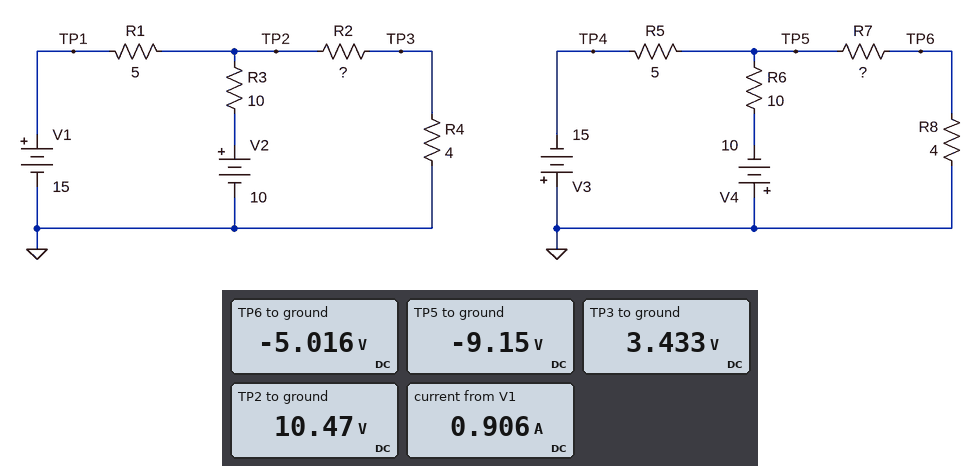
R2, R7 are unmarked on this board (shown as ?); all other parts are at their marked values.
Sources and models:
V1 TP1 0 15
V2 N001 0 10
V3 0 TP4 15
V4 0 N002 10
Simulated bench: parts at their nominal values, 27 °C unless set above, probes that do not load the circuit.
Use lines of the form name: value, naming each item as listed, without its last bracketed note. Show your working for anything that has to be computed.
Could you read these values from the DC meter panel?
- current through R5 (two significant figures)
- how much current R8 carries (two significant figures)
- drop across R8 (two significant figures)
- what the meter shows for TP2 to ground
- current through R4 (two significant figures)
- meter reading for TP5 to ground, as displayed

current through R5: (-9.15 V - (-15 V)) / 5 Ω = 1.2 A
how much current R8 carries: (0 V - (-5.016 V)) / 4 Ω = 1.3 A
drop across R8: 0 V - (-5.016 V) = 5.0 V
what the meter shows for TP2 to ground: 10.47 V
current through R4: (3.433 V) / 4 Ω = 860 mA
meter reading for TP5 to ground, as displayed: -9.15 V
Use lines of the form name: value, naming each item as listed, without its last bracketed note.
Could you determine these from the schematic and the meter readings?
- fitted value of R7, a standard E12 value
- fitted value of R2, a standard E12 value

fitted value of R7, a standard E12 value: 3.3 Ω
fitted value of R2, a standard E12 value: 8.2 Ω
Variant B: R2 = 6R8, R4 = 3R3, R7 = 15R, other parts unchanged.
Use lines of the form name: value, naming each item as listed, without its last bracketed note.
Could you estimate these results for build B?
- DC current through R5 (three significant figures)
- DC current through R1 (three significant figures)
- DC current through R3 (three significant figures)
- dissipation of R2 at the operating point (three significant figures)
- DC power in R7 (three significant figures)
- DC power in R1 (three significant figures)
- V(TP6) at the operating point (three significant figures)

DC current through R5: 731 mA
DC current through R1: 995 mA
DC current through R3: 2.48 mA
dissipation of R2 at the operating point: 6.70 W
DC power in R7: 5.35 W
DC power in R1: 4.95 W
V(TP6) at the operating point: -2.39 V
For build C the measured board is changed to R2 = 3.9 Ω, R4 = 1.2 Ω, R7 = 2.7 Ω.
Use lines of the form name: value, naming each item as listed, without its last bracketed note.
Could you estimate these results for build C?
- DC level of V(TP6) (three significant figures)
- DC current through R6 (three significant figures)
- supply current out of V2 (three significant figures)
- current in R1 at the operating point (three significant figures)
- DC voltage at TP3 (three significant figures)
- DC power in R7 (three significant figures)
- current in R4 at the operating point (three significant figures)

DC level of V(TP6): -5.32 V
DC current through R6: 110 mA
supply current out of V2: 194 mA
current in R1 at the operating point: 1.39 A
DC voltage at TP3: 1.90 V
DC power in R7: 4.77 W
current in R4 at the operating point: 1.58 A
